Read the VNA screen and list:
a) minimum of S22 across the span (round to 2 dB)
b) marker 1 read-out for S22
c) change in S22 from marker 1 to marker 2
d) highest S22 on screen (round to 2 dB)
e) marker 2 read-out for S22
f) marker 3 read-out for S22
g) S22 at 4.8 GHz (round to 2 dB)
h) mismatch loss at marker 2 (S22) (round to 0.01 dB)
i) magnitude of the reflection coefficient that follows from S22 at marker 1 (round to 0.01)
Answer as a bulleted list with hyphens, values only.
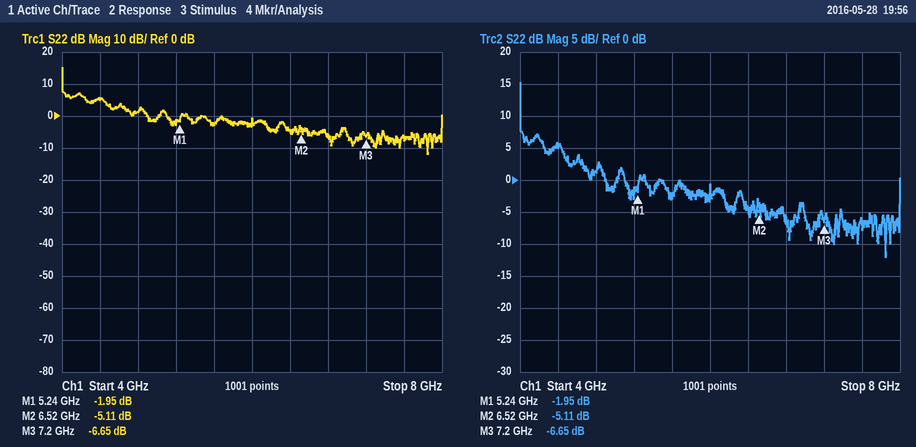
- -12 dB
- -1.95 dB
- -3.16 dB
- 16 dB
- -5.11 dB
- -6.65 dB
- 2 dB
- 1.60 dB
- 0.80
